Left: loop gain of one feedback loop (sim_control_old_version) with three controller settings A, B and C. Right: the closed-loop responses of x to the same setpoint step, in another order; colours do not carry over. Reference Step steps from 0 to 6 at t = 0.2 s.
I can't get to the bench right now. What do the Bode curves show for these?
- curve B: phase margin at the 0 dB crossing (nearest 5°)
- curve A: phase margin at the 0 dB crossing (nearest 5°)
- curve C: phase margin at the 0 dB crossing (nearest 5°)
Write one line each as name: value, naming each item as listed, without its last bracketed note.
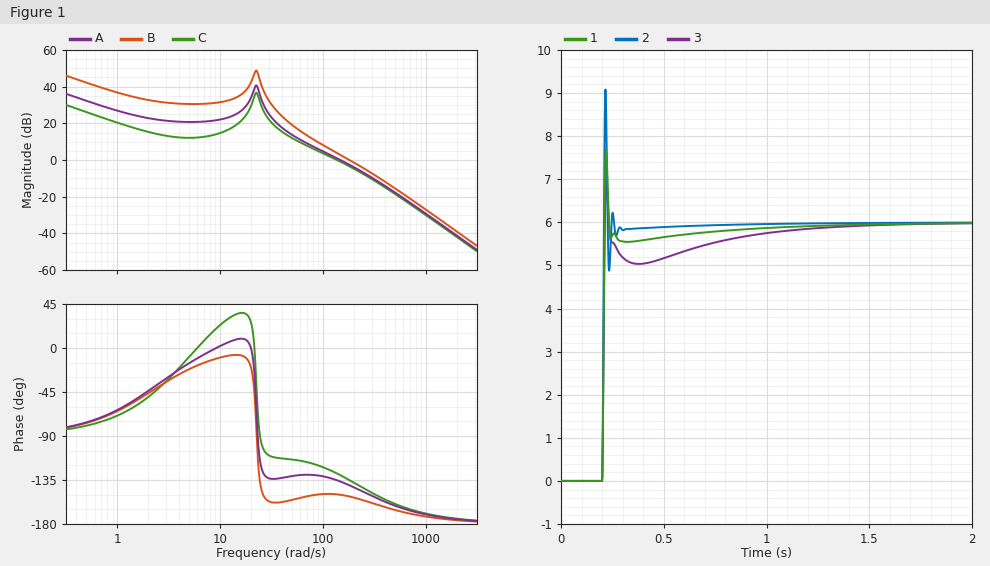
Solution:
curve B: phase margin at the 0 dB crossing: 30°
curve A: phase margin at the 0 dB crossing: 45°
curve C: phase margin at the 0 dB crossing: 50°
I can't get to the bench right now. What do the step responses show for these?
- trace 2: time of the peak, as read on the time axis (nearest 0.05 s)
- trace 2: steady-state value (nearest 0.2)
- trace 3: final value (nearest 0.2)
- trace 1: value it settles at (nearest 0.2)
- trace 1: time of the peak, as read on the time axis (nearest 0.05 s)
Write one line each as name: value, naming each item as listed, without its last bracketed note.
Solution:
trace 2: time of the peak, as read on the time axis: 0.20 s
trace 2: steady-state value: 6.0
trace 3: final value: 6.0
trace 1: value it settles at: 6.0
trace 1: time of the peak, as read on the time axis: 0.20 s
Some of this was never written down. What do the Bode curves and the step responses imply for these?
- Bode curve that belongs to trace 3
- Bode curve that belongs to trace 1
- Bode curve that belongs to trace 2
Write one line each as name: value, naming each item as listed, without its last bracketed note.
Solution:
Bode curve that belongs to trace 3: C
Bode curve that belongs to trace 1: A
Bode curve that belongs to trace 2: B
